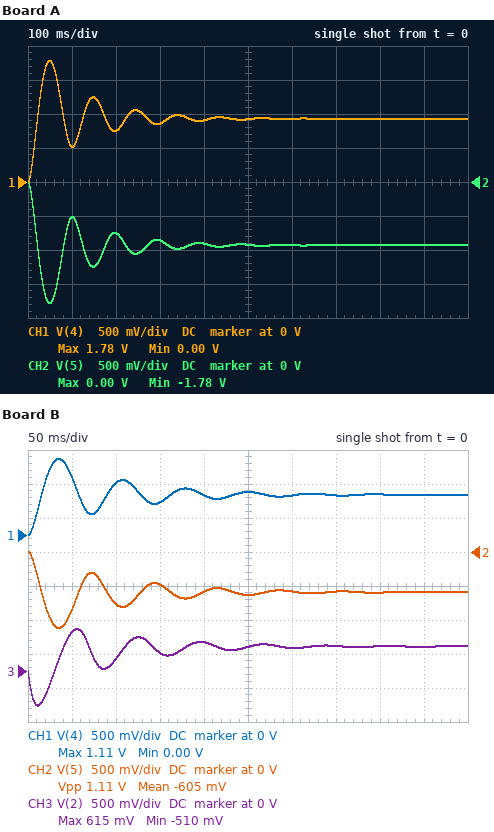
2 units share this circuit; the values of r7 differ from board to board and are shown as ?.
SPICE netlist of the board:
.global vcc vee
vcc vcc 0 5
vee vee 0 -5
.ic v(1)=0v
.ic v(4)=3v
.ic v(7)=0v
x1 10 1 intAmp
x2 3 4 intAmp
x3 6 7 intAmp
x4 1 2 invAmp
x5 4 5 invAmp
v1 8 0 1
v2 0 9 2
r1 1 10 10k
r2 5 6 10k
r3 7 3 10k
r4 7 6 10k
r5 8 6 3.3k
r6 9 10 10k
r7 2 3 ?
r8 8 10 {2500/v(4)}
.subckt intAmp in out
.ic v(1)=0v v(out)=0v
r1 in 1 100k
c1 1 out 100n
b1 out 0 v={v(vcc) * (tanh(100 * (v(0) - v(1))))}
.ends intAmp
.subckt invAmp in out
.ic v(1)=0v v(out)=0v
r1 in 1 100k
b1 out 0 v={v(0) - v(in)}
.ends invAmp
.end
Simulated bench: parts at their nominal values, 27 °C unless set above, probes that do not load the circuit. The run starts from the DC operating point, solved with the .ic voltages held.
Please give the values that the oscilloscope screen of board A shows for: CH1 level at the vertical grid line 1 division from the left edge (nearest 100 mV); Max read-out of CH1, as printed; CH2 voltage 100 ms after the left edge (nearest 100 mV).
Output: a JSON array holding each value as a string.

["500 mV", "1.78 V", "-500 mV"]
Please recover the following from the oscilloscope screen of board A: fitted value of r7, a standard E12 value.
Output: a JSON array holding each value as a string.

["8.2 kΩ"]
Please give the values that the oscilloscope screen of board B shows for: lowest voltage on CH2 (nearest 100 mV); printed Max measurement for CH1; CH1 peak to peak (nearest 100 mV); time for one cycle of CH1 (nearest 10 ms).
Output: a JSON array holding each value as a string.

["-1.1 V", "1.11 V", "1.1 V", "70 ms"]
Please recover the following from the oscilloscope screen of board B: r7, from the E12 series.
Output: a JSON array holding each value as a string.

["1.5 kΩ"]
